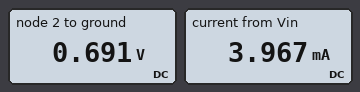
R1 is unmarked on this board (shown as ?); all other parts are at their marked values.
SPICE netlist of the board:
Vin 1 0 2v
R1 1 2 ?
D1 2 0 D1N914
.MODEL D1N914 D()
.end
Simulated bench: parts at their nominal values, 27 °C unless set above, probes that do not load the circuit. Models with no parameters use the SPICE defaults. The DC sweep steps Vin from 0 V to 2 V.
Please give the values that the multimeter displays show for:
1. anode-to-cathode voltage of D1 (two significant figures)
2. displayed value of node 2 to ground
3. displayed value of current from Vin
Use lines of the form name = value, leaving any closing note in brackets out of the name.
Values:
anode-to-cathode voltage of D1 = 690 mV
displayed value of node 2 to ground = 0.691 V
displayed value of current from Vin = 3.967 mA
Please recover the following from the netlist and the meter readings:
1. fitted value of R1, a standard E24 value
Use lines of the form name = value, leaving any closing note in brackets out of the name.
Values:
fitted value of R1, a standard E24 value = 330 Ω
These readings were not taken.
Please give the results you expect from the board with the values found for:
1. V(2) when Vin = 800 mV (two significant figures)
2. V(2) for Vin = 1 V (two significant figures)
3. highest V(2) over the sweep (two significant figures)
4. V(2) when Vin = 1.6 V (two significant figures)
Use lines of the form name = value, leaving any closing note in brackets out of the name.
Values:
V(2) when Vin = 800 mV = 640 mV
V(2) for Vin = 1 V = 660 mV
highest V(2) over the sweep = 690 mV
V(2) when Vin = 1.6 V = 680 mV
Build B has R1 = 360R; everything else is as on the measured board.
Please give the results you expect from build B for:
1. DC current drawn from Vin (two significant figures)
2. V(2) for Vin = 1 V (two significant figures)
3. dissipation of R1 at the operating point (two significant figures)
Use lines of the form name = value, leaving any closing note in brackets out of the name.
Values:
DC current drawn from Vin = 3.6 mA
V(2) for Vin = 1 V = 650 mV
dissipation of R1 at the operating point = 4.8 mW
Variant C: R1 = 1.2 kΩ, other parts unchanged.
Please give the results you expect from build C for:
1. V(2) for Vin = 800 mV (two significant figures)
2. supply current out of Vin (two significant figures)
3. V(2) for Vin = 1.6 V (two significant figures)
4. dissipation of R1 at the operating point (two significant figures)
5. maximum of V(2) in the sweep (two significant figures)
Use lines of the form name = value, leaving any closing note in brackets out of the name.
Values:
V(2) for Vin = 800 mV = 610 mV
supply current out of Vin = 1.1 mA
V(2) for Vin = 1.6 V = 650 mV
dissipation of R1 at the operating point = 1.5 mW
maximum of V(2) in the sweep = 660 mV
